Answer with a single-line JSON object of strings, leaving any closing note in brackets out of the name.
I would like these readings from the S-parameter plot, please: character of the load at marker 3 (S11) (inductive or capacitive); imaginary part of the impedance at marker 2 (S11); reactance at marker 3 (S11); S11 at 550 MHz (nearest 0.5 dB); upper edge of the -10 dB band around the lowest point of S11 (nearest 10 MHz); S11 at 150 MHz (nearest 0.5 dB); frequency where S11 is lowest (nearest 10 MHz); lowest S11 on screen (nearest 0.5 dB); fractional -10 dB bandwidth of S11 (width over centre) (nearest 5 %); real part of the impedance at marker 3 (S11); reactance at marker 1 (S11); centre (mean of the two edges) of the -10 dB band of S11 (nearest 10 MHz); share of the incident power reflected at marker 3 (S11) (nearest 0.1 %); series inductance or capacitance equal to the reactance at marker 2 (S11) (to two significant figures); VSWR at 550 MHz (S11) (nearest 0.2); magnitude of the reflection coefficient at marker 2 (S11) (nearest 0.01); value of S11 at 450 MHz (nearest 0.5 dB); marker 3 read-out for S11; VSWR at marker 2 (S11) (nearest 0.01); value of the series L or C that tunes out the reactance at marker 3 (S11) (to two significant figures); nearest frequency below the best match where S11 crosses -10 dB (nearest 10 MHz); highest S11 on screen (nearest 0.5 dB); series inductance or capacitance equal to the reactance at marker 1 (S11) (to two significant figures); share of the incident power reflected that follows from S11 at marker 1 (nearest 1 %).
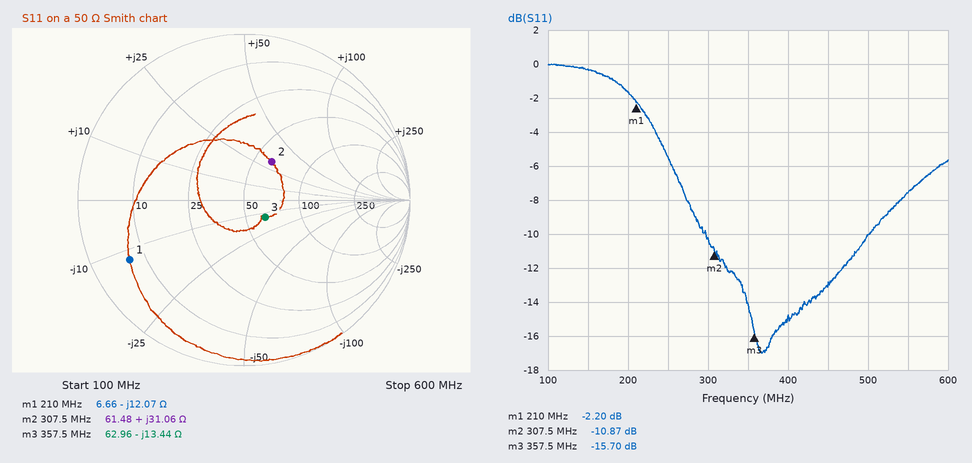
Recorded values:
{"character of the load at marker 3 (S11)": "capacitive", "imaginary part of the impedance at marker 2": "+31.06 Ω", "reactance at marker 3": "-13.44 Ω", "S11 at 550 MHz": "-7.5 dB", "upper edge of the -10 dB band around the lowest point of S11": "500 MHz", "S11 at 150 MHz": "-0.5 dB", "frequency where S11 is lowest": "370 MHz", "lowest S11 on screen": "-17.0 dB", "fractional -10 dB bandwidth of S11 (width over centre)": "50 %", "real part of the impedance at marker 3": "62.96 Ω", "reactance at marker 1": "-12.07 Ω", "centre (mean of the two edges) of the -10 dB band of S11": "400 MHz", "share of the incident power reflected at marker 3 (S11)": "2.7 %", "series inductance or capacitance equal to the reactance at marker 2 (S11)": "16 nH", "VSWR at 550 MHz (S11)": "2.4", "magnitude of the reflection coefficient at marker 2 (S11)": "0.29", "value of S11 at 450 MHz": "-13.0 dB", "marker 3 read-out for S11": "-15.70 dB", "VSWR at marker 2 (S11)": "1.80", "value of the series L or C that tunes out the reactance at marker 3 (S11)": "6.0 nH", "nearest frequency below the best match where S11 crosses -10 dB": "300 MHz", "highest S11 on screen": "0.0 dB", "series inductance or capacitance equal to the reactance at marker 1 (S11)": "63 pF", "share of the incident power reflected that follows from S11 at marker 1": "60 %"}
